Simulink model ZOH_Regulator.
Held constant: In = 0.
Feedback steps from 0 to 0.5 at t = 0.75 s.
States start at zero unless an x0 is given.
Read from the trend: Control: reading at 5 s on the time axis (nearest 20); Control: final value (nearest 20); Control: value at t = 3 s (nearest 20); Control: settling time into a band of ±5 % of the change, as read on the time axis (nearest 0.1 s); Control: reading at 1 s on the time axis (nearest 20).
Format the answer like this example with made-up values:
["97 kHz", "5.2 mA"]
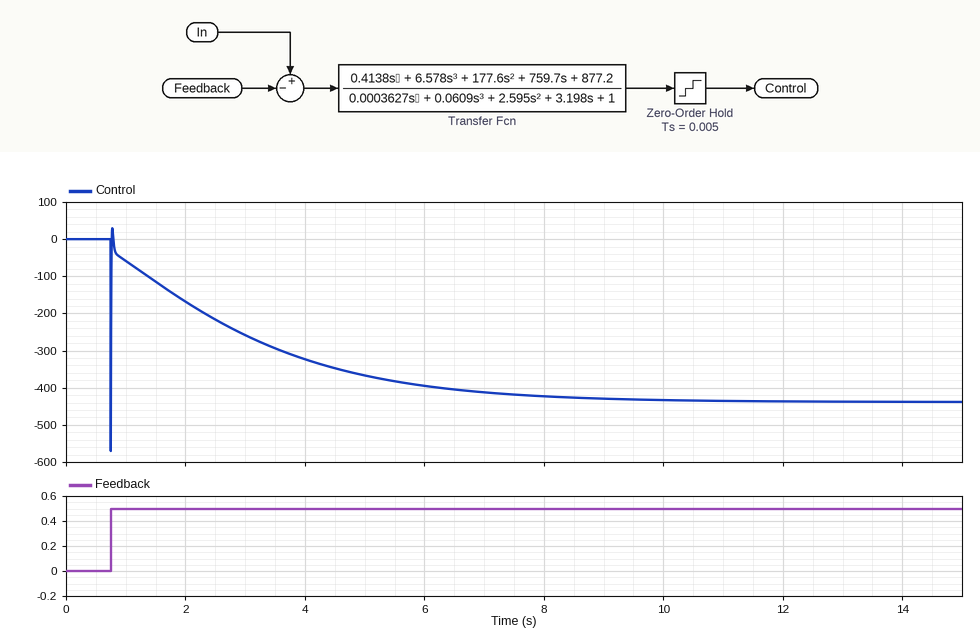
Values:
["-360", "-440", "-260", "7.3 s", "-60"]
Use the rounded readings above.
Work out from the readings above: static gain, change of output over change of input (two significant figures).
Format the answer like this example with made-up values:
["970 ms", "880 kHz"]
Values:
["-880"]
